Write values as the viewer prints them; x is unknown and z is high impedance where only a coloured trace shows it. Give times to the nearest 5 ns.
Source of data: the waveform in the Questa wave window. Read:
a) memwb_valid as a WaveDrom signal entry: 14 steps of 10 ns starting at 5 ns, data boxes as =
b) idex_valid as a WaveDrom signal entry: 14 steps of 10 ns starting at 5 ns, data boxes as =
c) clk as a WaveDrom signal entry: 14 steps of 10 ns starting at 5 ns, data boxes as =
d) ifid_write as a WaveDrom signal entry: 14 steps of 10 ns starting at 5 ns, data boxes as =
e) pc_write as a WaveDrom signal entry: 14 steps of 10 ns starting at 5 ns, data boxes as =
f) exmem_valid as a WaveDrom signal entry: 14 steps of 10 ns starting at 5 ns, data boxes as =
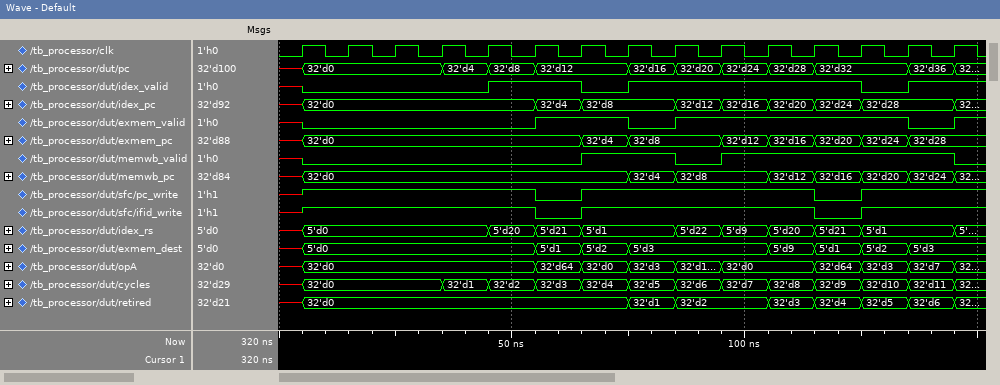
{name: 'memwb_valid', wave: '0.....1.01....'}
{name: 'idex_valid', wave: '0...1.01....01'}
{name: 'clk', wave: 'p.............'}
{name: 'ifid_write', wave: '1....01....01.'}
{name: 'pc_write', wave: '1....01....01.'}
{name: 'exmem_valid', wave: '0....1.01....0'}
